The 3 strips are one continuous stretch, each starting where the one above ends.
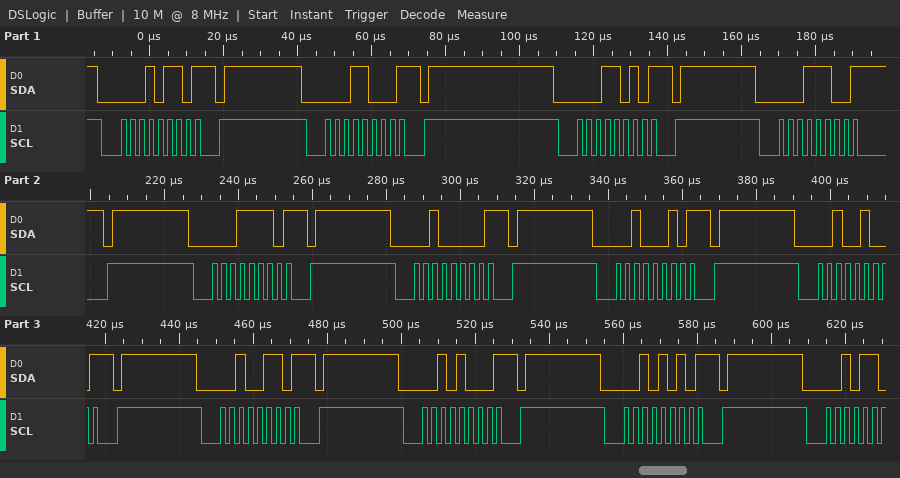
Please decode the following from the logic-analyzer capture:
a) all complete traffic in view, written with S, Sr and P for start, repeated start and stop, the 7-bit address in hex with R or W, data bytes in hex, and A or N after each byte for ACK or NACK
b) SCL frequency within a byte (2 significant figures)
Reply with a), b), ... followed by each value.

a) S 0BW N P S 0CW N P S 0DW N P S 0EW N P S 0FW N P S 10W N P S 11W N P S 12W N P S 13W N P S 14W N P S 15W N P
b) 400 kHz
